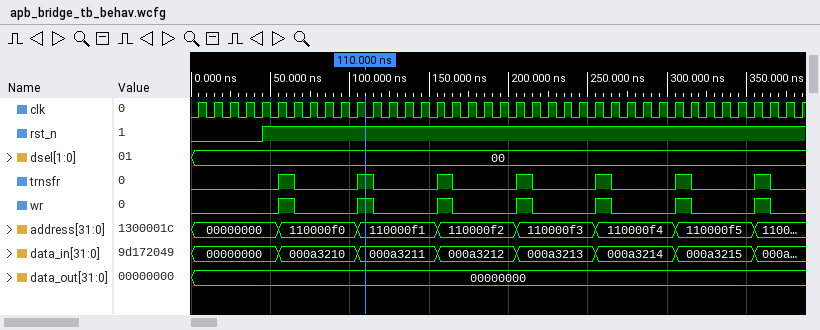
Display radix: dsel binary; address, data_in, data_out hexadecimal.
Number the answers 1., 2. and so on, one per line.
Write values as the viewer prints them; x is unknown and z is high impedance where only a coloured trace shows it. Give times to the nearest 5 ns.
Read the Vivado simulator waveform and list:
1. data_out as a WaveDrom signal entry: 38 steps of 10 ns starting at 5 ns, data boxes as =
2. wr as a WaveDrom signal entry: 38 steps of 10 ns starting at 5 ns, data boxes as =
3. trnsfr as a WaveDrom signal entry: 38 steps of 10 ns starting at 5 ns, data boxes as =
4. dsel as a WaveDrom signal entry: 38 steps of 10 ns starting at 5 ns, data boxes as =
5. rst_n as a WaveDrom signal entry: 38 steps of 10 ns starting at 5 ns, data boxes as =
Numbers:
1. {name: 'data_out', wave: '=.....................................', data: '00000000'}
2. {name: 'wr', wave: '0....10...10...10...10...10...10...10.'}
3. {name: 'trnsfr', wave: '0....10...10...10...10...10...10...10.'}
4. {name: 'dsel', wave: '=.....................................', data: '00'}
5. {name: 'rst_n', wave: '0...1.................................'}
